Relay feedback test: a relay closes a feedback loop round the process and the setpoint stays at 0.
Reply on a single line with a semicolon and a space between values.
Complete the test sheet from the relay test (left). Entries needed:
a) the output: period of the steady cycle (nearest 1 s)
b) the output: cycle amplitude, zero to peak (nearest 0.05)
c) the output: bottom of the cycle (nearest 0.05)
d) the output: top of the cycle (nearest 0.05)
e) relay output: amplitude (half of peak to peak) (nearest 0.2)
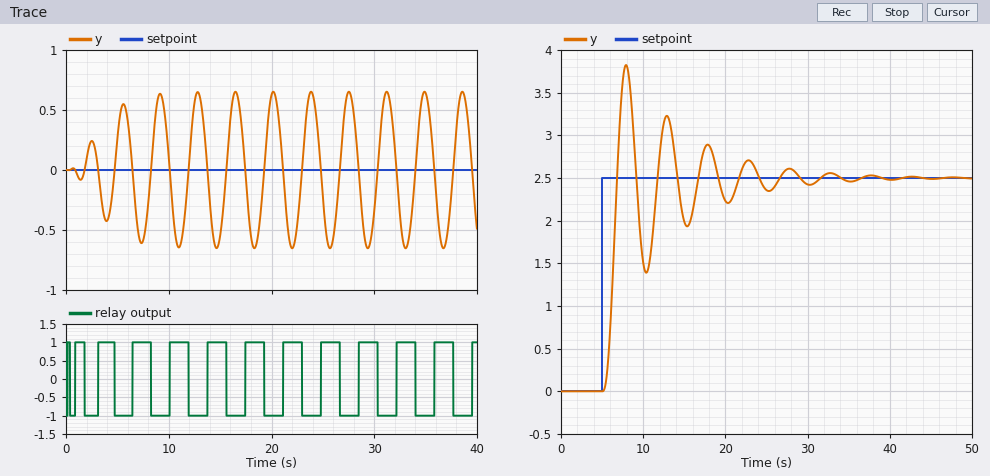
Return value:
4 s; 0.65; -0.65; 0.65; 1.0
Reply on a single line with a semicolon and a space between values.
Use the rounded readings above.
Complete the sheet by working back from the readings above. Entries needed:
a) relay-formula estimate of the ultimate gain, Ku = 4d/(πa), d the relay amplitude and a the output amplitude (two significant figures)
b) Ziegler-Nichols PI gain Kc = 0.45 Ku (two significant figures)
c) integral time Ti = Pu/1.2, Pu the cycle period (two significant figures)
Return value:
2.0; 0.90; 3.3 s
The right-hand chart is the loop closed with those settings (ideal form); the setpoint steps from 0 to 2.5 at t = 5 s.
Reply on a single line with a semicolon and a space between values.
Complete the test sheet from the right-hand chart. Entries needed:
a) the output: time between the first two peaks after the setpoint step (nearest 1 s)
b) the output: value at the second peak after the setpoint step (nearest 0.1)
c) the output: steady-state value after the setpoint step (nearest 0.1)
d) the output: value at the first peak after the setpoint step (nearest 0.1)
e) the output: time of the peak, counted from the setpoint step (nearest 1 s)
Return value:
5 s; 3.2; 2.5; 3.8; 3 s
